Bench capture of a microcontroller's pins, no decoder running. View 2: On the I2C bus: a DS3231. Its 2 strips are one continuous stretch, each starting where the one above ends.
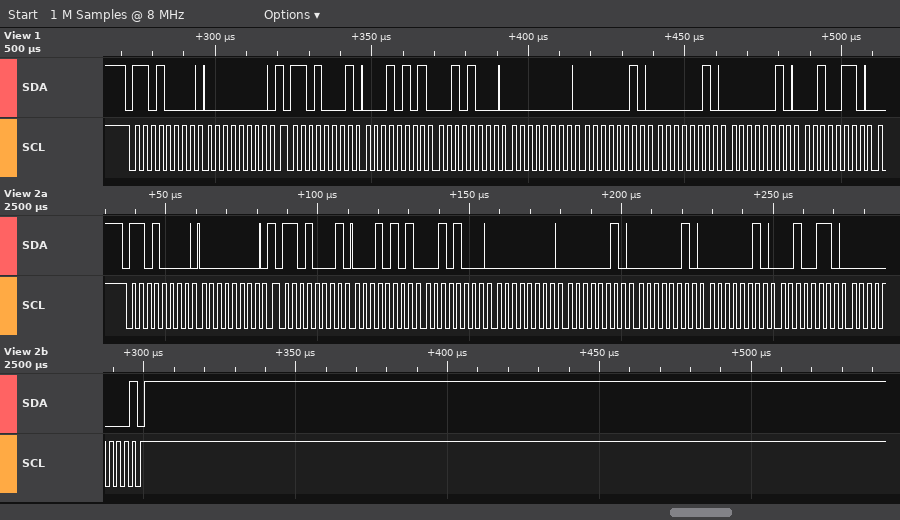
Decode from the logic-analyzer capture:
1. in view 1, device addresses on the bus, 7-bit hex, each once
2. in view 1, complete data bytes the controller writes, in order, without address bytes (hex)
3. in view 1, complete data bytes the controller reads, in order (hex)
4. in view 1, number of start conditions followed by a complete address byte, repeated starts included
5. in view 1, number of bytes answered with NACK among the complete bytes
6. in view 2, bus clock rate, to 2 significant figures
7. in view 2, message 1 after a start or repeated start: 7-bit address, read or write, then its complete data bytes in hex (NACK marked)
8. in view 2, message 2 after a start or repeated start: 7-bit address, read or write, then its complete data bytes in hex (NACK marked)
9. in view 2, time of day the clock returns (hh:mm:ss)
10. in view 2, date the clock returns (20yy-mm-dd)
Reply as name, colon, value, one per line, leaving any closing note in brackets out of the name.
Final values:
in view 1, device addresses on the bus, 7-bit hex, each once: 0x68
in view 1, complete data bytes the controller writes, in order, without address bytes: 00
in view 1, complete data bytes the controller reads, in order: 15 28 00 02 02 02 26
in view 1, number of start conditions followed by a complete address byte, repeated starts included: 2
in view 1, number of bytes answered with NACK among the complete bytes: 0
in view 2, bus clock rate, to 2 significant figures: 400 kHz
in view 2, message 1 after a start or repeated start: 7-bit address, read or write, then its complete data bytes in hex: 0x68 write: 00
in view 2, message 2 after a start or repeated start: 7-bit address, read or write, then its complete data bytes in hex: 0x68 read: 15 28 00 02 02 02 26 00 NACK
in view 2, time of day the clock returns: 00:28:15
in view 2, date the clock returns: 2026-02-02
